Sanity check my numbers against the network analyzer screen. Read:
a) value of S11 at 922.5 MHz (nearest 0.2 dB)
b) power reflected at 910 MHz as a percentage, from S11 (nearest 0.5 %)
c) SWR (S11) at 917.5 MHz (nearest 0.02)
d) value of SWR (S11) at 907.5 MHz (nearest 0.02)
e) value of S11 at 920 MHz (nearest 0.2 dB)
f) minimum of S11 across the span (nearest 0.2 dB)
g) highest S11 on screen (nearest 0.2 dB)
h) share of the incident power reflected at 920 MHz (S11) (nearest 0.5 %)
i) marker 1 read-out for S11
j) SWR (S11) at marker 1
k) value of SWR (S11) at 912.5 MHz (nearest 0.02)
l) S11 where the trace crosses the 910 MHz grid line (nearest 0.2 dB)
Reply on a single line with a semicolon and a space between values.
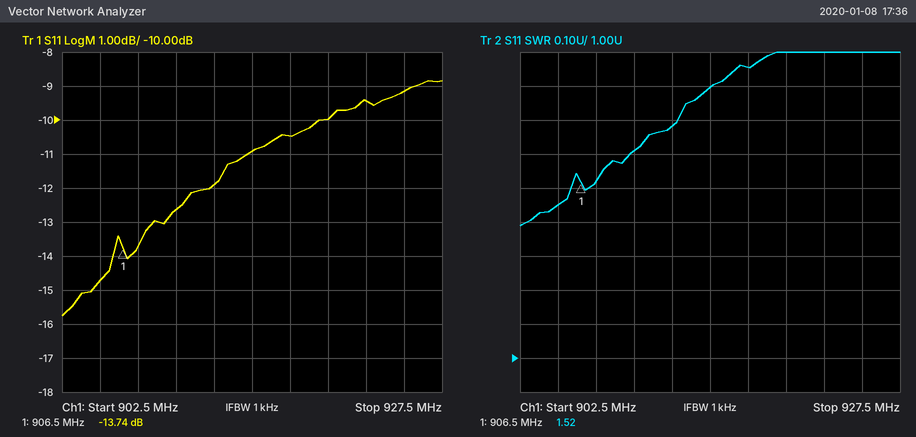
-9.4 dB; 5.5 %; 1.86; 1.52; -10.0 dB; -15.8 dB; -8.8 dB; 10.0 %; -13.74 dB; 1.52; 1.68; -12.6 dB
